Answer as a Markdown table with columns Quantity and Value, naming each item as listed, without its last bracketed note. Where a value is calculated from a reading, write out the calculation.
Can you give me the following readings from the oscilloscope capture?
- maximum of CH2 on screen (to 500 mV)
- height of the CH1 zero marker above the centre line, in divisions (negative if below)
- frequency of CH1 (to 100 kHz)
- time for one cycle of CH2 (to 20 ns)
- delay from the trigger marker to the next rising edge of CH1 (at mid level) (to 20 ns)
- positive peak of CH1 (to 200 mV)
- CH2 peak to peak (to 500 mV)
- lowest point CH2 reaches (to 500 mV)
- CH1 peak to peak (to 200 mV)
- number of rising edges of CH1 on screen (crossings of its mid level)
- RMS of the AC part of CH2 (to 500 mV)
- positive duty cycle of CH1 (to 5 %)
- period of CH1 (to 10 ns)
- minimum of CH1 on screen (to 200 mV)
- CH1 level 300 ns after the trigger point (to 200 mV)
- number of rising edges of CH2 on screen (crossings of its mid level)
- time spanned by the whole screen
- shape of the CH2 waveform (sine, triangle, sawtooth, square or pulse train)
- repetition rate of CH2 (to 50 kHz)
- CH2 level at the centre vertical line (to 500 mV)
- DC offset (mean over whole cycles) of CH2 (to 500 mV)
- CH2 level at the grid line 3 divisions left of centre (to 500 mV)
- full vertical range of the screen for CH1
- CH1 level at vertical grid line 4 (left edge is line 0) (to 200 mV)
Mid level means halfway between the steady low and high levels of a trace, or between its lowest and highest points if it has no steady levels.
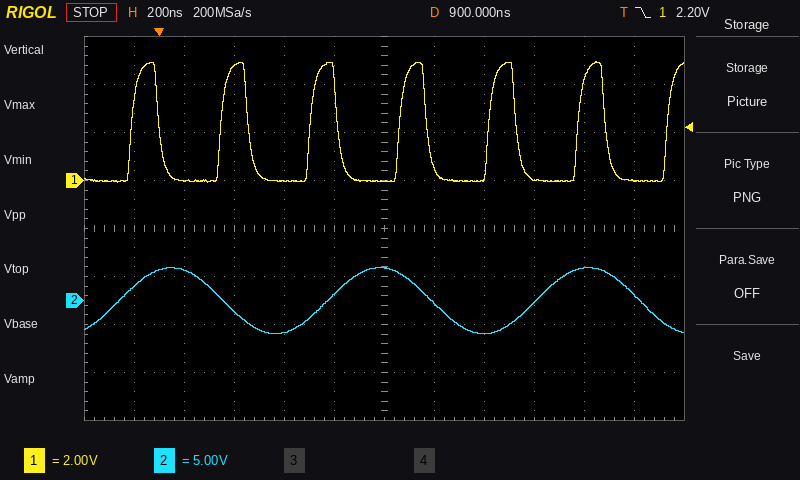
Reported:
| Quantity | Value |
|---|---|
| maximum of CH2 on screen | 3.5 V |
| height of the CH1 zero marker above the centre line, in divisions | +1.0 div |
| frequency of CH1 | 1 / 360 ns ≈ 2.8 MHz |
| time for one cycle of CH2 | 840 ns |
| delay from the trigger marker to the next rising edge of CH1 (at mid level) | 240 ns |
| positive peak of CH1 | 5.0 V |
| CH2 peak to peak | 3.5 V − (-3.5 V) = 7.0 V |
| lowest point CH2 reaches | -3.5 V |
| CH1 peak to peak | 5.0 V − (0.0 V) = 5.0 V |
| number of rising edges of CH1 on screen | 7 |
| RMS of the AC part of CH2 | 7.0 V / (2√2) ≈ 2.5 V |
| positive duty cycle of CH1 | 30 % |
| period of CH1 | 360 ns |
| minimum of CH1 on screen | 0.0 V |
| CH1 level 300 ns after the trigger point | 4.8 V |
| number of rising edges of CH2 on screen | 3 |
| time spanned by the whole screen | 2.4 µs |
| shape of the CH2 waveform | sine |
| repetition rate of CH2 | 1 / 840 ns ≈ 1.19 MHz, so 1.20 MHz to the nearest 50 kHz |
| CH2 level at the centre vertical line | 3.5 V |
| DC offset (mean over whole cycles) of CH2 | (3.5 V + (-3.5 V)) / 2 ≈ 0.0 V |
| CH2 level at the grid line 3 divisions left of centre | -1.0 V |
| full vertical range of the screen for CH1 | 16 V |
| CH1 level at vertical grid line 4 (left edge is line 0) | 0.0 V |
